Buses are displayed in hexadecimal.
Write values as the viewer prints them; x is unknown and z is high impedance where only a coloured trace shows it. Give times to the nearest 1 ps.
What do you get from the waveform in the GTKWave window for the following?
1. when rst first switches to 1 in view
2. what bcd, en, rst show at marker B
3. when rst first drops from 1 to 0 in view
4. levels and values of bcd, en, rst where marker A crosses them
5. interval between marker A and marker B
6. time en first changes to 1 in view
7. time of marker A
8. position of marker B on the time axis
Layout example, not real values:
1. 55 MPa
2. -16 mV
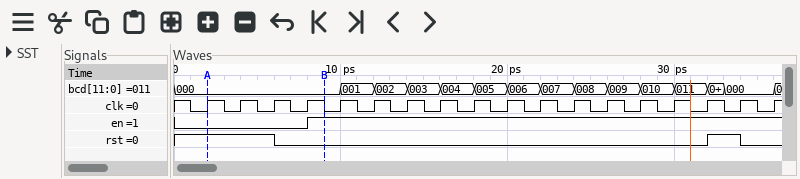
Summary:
1. 32 ps
2. bcd=000, en=1, rst=0
3. 6 ps
4. bcd=000, en=0, rst=1
5. 7 ps
6. 8 ps
7. 2 ps
8. 9 ps
